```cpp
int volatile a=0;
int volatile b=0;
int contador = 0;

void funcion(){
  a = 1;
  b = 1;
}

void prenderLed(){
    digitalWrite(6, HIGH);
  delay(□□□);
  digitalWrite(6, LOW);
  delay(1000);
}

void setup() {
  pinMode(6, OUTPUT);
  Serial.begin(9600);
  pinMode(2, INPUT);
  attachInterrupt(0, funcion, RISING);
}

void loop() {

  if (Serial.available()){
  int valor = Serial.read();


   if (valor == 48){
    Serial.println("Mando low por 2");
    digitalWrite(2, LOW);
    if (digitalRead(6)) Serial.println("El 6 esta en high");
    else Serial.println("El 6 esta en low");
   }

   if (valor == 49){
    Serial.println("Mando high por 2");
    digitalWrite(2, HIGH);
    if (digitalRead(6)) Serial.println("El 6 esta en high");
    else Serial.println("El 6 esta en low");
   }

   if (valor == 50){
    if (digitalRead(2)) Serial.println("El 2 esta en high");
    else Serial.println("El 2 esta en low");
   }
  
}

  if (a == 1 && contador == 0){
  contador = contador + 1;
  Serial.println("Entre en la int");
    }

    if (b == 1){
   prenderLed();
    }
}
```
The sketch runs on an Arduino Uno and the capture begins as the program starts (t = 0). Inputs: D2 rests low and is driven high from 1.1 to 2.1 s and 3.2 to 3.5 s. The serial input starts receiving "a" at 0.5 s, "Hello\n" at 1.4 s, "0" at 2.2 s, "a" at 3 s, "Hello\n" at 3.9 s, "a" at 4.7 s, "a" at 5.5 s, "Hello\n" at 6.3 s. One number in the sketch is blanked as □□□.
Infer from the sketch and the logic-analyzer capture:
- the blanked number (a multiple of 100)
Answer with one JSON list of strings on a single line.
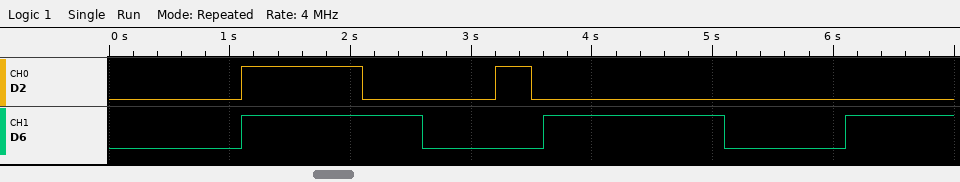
["1500"]
